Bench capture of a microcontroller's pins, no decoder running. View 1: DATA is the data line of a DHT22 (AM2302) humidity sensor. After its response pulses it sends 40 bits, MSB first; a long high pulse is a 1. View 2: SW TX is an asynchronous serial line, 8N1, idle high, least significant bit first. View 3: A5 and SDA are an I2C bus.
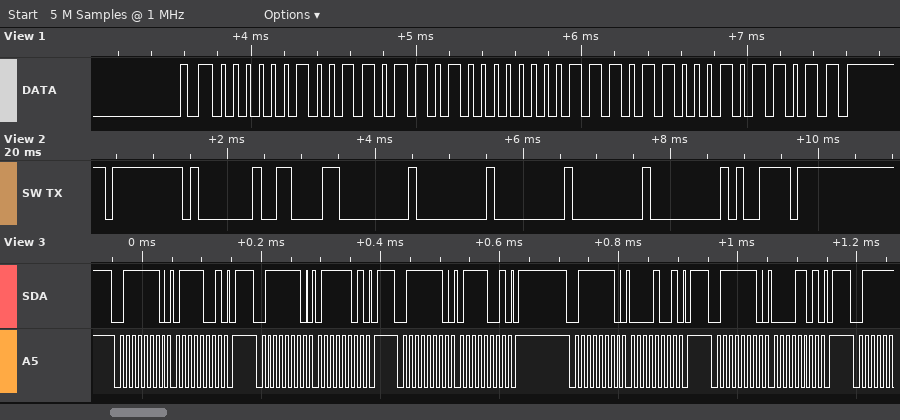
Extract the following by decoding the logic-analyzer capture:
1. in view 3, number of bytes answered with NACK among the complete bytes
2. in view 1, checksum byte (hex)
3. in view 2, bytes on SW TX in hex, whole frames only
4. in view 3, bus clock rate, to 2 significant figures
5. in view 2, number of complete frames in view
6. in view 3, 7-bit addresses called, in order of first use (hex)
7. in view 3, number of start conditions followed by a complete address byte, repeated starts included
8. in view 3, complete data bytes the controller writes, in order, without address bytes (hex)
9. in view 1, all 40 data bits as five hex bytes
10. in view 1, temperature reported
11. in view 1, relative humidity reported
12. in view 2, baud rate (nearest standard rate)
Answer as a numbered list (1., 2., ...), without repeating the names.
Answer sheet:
1. 0
2. 0x5B
3. FF 01 86 00 00 00 00 00 79
4. 100 kHz
5. 9
6. 0x3F
7. 5
8. 79 7D 79 09 0D
9. 02 6D 00 EC 5B
10. 23.6 °C
11. 62.1 %
12. 9600 baud
